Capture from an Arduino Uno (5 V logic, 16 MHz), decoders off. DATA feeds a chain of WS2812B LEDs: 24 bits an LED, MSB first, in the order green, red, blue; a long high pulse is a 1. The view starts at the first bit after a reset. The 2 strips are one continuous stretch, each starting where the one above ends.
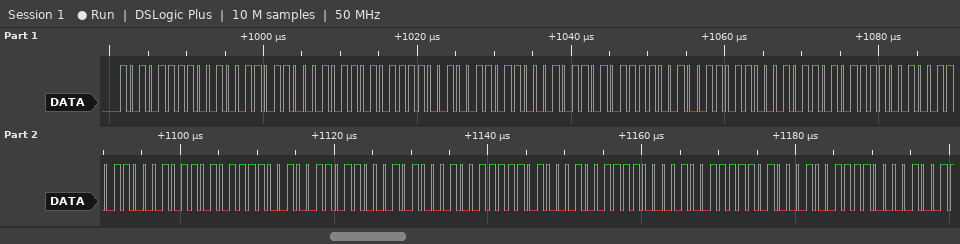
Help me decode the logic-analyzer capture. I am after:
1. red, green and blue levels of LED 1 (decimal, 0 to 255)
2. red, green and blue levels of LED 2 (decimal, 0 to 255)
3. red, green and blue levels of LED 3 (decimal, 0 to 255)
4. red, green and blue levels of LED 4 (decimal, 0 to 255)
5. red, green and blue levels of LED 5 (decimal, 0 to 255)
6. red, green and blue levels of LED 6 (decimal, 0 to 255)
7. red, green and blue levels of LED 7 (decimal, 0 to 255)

38, 175, 197
38, 175, 197
38, 175, 197
38, 175, 197
38, 175, 197
232, 19, 158
232, 19, 158
